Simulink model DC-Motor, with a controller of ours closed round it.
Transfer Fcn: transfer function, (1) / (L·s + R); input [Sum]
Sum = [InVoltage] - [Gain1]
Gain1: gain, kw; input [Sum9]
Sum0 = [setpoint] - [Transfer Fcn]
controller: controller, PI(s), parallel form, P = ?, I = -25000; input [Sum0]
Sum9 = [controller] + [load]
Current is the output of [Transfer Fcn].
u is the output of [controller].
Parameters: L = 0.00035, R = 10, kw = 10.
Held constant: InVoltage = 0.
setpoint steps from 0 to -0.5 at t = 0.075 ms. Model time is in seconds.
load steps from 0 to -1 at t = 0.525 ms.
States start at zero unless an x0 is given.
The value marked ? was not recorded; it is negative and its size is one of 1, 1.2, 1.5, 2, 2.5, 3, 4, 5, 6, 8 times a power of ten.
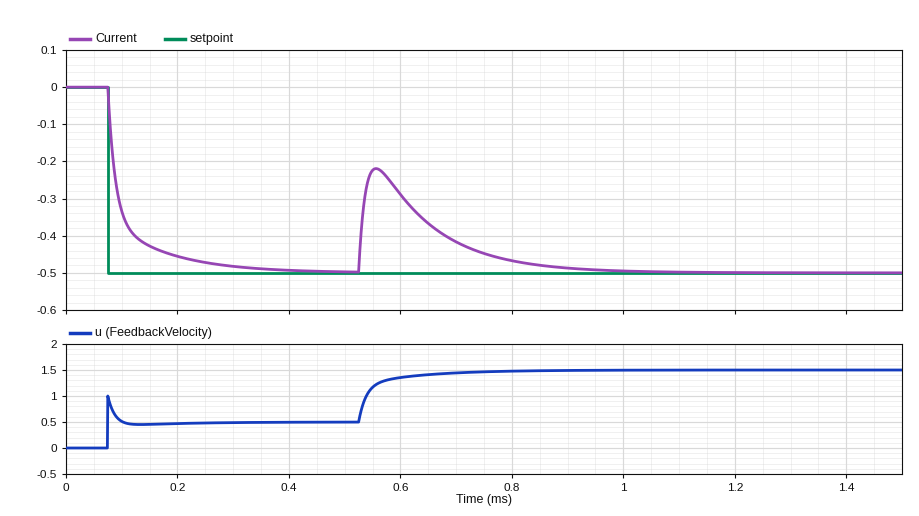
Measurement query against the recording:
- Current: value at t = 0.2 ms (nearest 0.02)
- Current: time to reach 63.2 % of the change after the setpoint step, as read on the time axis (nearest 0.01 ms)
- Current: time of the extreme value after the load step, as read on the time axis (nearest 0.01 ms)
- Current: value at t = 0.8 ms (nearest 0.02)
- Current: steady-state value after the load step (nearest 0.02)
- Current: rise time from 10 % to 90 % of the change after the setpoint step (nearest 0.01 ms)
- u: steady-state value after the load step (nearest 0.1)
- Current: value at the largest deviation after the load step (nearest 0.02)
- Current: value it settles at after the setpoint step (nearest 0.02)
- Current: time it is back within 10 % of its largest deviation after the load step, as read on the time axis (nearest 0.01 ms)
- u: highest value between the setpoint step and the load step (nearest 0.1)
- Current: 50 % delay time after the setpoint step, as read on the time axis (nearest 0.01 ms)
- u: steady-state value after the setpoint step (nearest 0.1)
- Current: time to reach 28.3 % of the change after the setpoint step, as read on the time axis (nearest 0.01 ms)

-0.46
0.10 ms
0.56 ms
-0.46
-0.50
0.11 ms
1.5
-0.22
-0.50
0.82 ms
1.0
0.09 ms
0.5
0.08 ms
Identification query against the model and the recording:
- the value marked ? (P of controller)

-2
